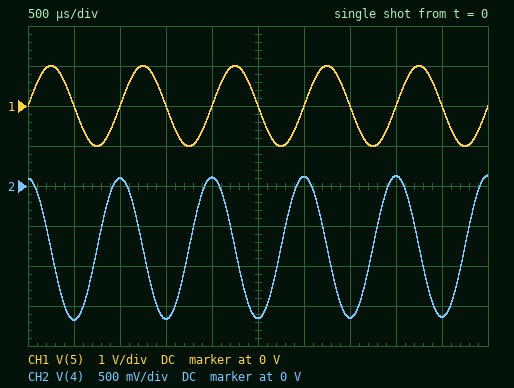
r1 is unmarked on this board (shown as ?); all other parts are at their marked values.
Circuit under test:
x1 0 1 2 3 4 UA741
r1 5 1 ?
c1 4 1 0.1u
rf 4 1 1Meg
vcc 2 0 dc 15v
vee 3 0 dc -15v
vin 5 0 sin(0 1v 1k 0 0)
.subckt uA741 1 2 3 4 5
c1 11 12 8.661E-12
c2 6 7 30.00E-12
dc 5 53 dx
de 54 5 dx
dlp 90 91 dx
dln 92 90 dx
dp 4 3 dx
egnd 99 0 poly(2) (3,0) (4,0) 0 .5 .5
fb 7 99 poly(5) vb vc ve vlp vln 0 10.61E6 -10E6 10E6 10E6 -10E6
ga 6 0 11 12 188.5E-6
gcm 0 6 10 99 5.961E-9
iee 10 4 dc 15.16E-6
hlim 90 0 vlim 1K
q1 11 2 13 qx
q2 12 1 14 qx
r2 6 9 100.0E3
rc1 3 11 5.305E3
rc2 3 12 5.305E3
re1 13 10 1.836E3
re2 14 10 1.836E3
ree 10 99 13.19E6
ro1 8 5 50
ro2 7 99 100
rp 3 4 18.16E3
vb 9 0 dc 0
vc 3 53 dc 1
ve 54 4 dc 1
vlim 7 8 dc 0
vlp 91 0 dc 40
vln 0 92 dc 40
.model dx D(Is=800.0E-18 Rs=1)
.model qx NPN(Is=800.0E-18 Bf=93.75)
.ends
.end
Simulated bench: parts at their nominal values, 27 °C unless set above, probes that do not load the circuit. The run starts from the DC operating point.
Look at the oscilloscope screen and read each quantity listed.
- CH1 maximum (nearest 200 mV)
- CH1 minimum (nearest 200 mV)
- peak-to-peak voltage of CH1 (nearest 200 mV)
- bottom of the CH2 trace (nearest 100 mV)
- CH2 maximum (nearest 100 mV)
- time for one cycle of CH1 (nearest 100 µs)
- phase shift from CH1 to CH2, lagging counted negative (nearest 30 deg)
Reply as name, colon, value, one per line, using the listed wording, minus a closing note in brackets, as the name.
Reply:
CH1 maximum: 1.0 V
CH1 minimum: -1.0 V
peak-to-peak voltage of CH1: 2.0 V
bottom of the CH2 trace: -1.7 V
CH2 maximum: 100 mV
time for one cycle of CH1: 1.0 ms
phase shift from CH1 to CH2, lagging counted negative: 90 deg
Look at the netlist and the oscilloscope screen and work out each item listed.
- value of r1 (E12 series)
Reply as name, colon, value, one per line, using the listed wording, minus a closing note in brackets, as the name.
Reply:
value of r1: 1.8 kΩ
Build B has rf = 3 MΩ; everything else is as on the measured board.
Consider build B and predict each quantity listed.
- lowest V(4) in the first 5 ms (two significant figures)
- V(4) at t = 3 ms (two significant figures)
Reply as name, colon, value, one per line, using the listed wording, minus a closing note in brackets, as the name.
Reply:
lowest V(4) in the first 5 ms: -1.5 V
V(4) at t = 3 ms: 280 mV
